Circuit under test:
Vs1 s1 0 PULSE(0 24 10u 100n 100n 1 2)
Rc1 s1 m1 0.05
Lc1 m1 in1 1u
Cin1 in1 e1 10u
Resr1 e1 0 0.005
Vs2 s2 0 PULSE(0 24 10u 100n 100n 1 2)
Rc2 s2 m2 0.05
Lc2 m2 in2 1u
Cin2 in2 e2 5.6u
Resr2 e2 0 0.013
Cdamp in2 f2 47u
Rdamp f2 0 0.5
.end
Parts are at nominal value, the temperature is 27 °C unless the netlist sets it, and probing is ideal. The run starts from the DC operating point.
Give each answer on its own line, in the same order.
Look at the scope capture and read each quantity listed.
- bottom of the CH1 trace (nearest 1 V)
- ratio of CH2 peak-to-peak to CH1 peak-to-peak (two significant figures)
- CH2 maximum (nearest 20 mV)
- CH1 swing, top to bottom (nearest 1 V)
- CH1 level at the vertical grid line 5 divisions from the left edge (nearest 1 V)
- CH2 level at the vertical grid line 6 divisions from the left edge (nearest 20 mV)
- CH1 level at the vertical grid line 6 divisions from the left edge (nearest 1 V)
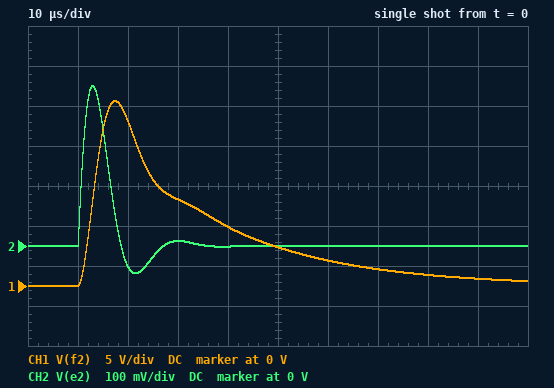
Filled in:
0 V
0.020
400 mV
23 V
5 V
0 V
3 V
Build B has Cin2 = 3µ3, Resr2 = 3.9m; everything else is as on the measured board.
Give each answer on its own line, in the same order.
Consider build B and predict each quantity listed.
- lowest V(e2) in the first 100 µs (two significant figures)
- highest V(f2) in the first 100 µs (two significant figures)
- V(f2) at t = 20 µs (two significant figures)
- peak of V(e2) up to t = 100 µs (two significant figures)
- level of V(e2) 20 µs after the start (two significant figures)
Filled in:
-8.2 mV
22 V
18 V
84 mV
-7.5 mV
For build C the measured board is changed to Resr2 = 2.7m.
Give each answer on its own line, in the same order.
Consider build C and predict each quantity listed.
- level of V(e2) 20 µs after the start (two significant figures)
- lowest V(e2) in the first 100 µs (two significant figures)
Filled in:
-12 mV
-15 mV
